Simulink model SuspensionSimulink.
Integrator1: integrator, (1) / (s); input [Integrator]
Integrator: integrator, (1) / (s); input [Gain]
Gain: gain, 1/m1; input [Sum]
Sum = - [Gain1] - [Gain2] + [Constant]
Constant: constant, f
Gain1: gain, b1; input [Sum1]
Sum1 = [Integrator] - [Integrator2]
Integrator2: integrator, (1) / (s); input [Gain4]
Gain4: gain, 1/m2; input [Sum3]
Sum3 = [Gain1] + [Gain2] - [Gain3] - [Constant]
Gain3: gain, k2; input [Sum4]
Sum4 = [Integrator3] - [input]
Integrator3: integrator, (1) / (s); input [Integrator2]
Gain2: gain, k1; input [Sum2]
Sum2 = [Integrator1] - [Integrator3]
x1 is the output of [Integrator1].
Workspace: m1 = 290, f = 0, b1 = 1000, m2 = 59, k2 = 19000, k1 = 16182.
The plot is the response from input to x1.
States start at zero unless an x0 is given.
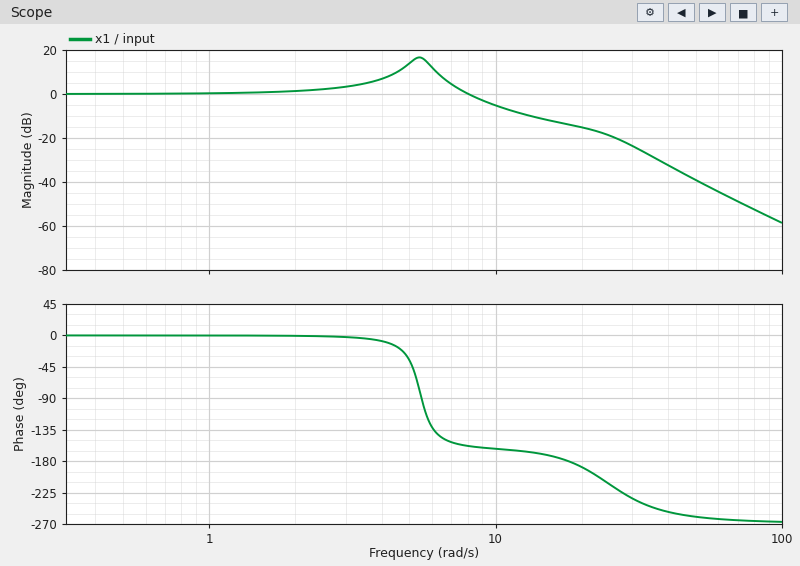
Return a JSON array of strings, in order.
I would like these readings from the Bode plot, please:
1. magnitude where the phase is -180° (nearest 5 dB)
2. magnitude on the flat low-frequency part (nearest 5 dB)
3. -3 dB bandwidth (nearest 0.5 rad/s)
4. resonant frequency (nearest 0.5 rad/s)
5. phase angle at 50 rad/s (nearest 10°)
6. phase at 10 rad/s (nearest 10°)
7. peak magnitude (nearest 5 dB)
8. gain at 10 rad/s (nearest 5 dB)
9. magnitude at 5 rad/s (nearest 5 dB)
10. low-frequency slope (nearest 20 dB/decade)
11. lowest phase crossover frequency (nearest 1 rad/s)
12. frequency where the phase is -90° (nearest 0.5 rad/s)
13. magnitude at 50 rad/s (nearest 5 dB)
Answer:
["-15 dB", "0 dB", "9.0 rad/s", "5.5 rad/s", "-260°", "-160°", "15 dB", "-5 dB", "15 dB", "0 dB/decade", "18 rad/s", "5.5 rad/s", "-40 dB"]
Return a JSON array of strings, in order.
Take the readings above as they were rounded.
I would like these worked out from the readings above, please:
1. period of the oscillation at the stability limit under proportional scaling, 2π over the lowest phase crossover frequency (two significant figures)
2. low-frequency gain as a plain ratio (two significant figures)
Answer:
["0.35 s", "1.0"]
